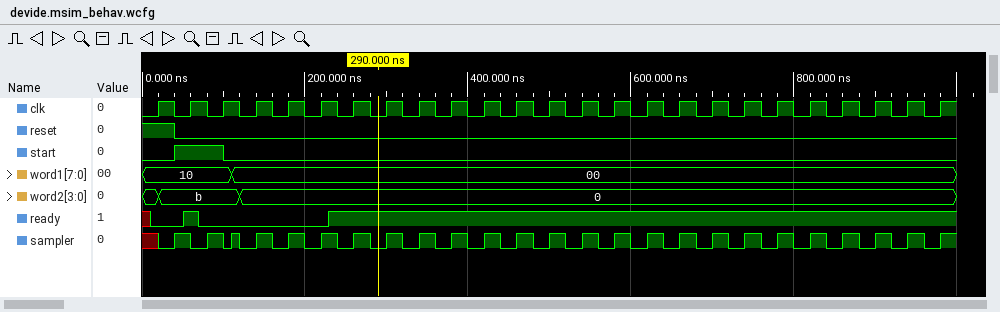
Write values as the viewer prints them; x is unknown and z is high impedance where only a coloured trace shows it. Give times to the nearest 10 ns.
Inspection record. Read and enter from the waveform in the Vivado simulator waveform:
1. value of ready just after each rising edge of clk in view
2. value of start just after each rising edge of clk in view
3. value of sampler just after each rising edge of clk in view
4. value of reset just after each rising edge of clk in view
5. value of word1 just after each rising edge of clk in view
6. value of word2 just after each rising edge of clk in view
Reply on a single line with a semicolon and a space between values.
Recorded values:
0 1 0 0 0 0 1 1 1 1 1 1 1 1 1 1 1 1 1 1 1 1 1 1 1; 0 1 0 0 0 0 0 0 0 0 0 0 0 0 0 0 0 0 0 0 0 0 0 0 0; 0 0 0 1 1 1 1 1 1 1 1 1 1 1 1 1 1 1 1 1 1 1 1 1 1; 1 0 0 0 0 0 0 0 0 0 0 0 0 0 0 0 0 0 0 0 0 0 0 0 0; 10, 10, 10, 00, 00, 00, 00, 00, 00, 00, 00, 00, 00, 00, 00, 00, 00, 00, 00, 00, 00, 00, 00, 00, 00; b, b, b, 0, 0, 0, 0, 0, 0, 0, 0, 0, 0, 0, 0, 0, 0, 0, 0, 0, 0, 0, 0, 0, 0
